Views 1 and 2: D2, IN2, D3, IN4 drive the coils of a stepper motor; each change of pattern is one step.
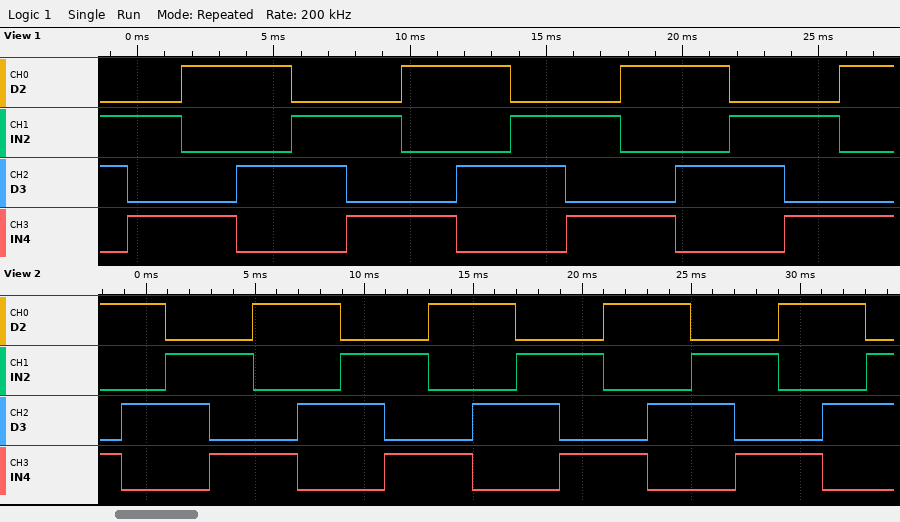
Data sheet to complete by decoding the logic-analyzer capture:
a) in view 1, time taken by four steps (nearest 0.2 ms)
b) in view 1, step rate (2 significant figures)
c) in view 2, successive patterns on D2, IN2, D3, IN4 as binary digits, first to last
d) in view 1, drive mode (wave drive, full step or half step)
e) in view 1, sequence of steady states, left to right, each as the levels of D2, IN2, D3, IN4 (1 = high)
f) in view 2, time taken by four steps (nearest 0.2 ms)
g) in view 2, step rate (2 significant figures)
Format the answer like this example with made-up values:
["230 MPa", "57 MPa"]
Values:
["8.0 ms", "500 steps/s", "1001 1010 0110 0101 1001 1010 0110 0101 1001 1010 0110 0101 1001 1010 0110 0101 1001 1010 0110", "full step", "0110 0101 1001 1010 0110 0101 1001 1010 0110 0101 1001 1010 0110 0101 1001", "8.0 ms", "500 steps/s"]
